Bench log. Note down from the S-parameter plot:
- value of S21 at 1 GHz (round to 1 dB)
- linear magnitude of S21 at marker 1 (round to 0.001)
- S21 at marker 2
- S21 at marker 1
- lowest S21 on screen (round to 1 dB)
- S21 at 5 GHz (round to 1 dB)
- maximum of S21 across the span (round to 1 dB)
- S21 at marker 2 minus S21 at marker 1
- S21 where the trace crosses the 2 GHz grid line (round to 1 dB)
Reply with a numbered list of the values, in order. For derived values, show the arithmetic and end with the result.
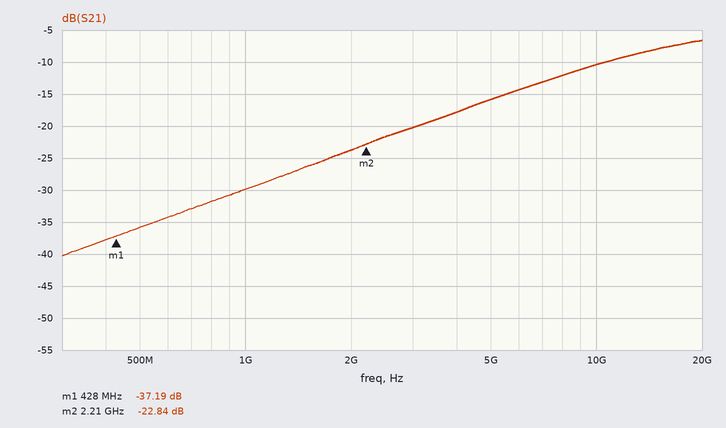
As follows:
1. -30 dB
2. 10^(-37.19/20) ≈ 0.014
3. -22.84 dB
4. -37.19 dB
5. -40 dB
6. -16 dB
7. -7 dB
8. -22.84 − (-37.19) = 14.35 dB
9. -24 dB
